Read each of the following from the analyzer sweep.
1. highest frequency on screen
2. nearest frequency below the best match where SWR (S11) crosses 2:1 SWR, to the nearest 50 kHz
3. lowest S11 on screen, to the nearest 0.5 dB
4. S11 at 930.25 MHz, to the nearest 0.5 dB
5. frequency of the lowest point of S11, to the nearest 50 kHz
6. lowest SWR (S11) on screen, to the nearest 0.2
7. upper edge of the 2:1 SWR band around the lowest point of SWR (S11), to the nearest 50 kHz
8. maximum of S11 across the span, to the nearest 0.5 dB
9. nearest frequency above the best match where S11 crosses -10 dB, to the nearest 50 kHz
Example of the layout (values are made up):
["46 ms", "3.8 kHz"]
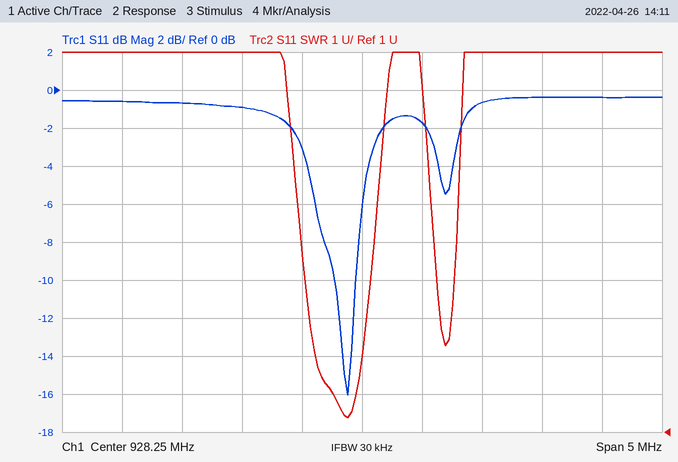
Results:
["930.75 MHz", "928.00 MHz", "-16.0 dB", "-0.5 dB", "928.15 MHz", "1.4", "928.20 MHz", "-0.5 dB", "928.20 MHz"]
